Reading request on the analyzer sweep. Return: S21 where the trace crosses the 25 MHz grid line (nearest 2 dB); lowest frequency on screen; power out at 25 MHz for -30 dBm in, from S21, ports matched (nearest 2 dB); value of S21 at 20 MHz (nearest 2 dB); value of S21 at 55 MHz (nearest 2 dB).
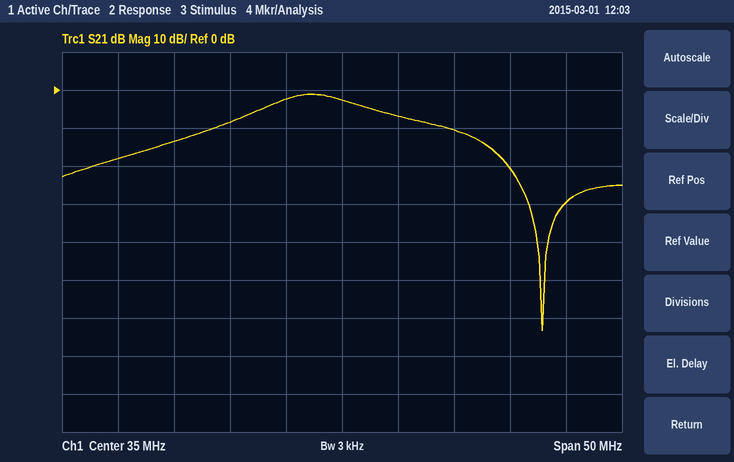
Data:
-8 dB
10 MHz
-38 dBm
-14 dB
-30 dB
